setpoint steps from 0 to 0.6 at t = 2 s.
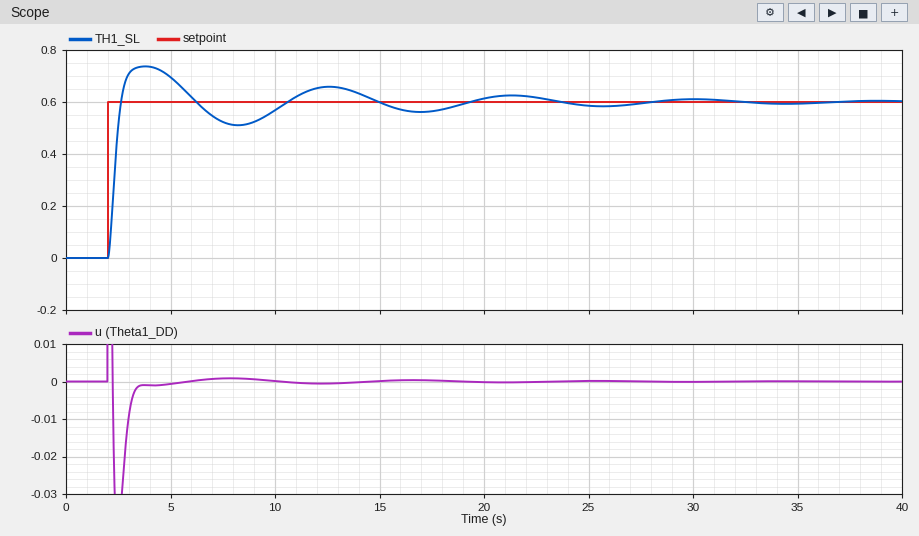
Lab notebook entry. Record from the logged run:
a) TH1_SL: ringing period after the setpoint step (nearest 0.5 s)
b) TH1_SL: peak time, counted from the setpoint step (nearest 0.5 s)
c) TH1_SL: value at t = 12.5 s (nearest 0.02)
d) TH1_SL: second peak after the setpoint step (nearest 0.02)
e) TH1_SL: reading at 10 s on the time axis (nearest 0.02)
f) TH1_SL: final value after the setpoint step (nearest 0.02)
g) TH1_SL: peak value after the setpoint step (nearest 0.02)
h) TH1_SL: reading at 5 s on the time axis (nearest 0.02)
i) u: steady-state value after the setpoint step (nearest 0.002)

9.0 s
2.0 s
0.66
0.66
0.56
0.60
0.74
0.70
0.000
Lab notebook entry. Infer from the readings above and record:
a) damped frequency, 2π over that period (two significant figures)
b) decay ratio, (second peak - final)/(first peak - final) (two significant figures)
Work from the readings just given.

0.70 rad/s
0.43
